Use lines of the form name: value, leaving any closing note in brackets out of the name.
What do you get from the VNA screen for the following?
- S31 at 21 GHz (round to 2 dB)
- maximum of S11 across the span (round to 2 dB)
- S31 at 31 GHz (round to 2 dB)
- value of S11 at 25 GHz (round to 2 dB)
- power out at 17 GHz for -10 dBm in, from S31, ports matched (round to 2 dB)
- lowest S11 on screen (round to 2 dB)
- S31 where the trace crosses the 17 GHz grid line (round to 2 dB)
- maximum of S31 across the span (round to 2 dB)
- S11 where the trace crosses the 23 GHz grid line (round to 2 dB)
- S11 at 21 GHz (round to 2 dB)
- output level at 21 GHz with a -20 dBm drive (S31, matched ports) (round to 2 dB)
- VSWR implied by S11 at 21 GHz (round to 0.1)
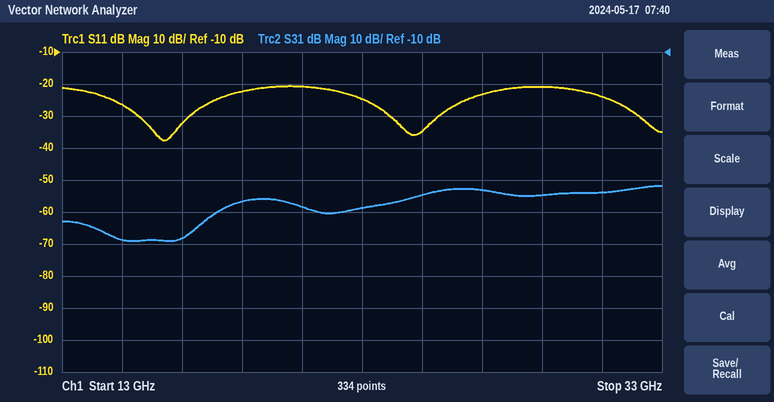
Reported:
S31 at 21 GHz: -58 dB
maximum of S11 across the span: -20 dB
S31 at 31 GHz: -54 dB
value of S11 at 25 GHz: -34 dB
power out at 17 GHz for -10 dBm in, from S31, ports matched: -78 dBm
lowest S11 on screen: -38 dB
S31 where the trace crosses the 17 GHz grid line: -68 dB
maximum of S31 across the span: -52 dB
S11 where the trace crosses the 23 GHz grid line: -24 dB
S11 at 21 GHz: -20 dB
output level at 21 GHz with a -20 dBm drive (S31, matched ports): -78 dBm
VSWR implied by S11 at 21 GHz: 1.2
